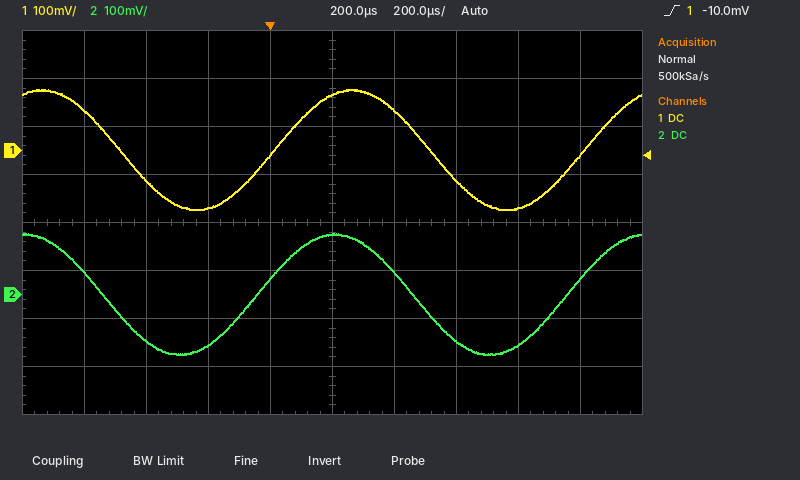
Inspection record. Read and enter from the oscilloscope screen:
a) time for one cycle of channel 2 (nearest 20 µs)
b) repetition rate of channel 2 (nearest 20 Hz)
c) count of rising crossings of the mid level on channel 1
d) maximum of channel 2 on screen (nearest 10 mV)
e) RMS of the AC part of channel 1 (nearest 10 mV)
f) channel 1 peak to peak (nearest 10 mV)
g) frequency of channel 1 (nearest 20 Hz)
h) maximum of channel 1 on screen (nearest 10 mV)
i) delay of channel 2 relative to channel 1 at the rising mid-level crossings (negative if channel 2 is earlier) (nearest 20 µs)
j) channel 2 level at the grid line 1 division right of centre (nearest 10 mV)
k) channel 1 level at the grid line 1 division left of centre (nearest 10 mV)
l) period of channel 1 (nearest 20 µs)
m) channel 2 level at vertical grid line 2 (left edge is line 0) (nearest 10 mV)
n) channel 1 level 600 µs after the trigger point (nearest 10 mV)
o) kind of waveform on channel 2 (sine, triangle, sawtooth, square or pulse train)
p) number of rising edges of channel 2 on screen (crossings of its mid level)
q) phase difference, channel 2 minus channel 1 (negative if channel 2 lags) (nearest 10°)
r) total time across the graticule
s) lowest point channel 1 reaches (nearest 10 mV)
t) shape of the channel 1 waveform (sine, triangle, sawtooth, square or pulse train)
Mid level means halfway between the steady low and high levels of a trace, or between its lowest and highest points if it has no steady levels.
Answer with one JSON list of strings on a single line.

["1.00 ms", "1.00 kHz", "2", "130 mV", "90 mV", "250 mV", "1.00 kHz", "130 mV", "-60 µs", "50 mV", "-10 mV", "1.00 ms", "-100 mV", "-60 mV", "sine", "2", "+20°", "2 ms", "-120 mV", "sine"]
